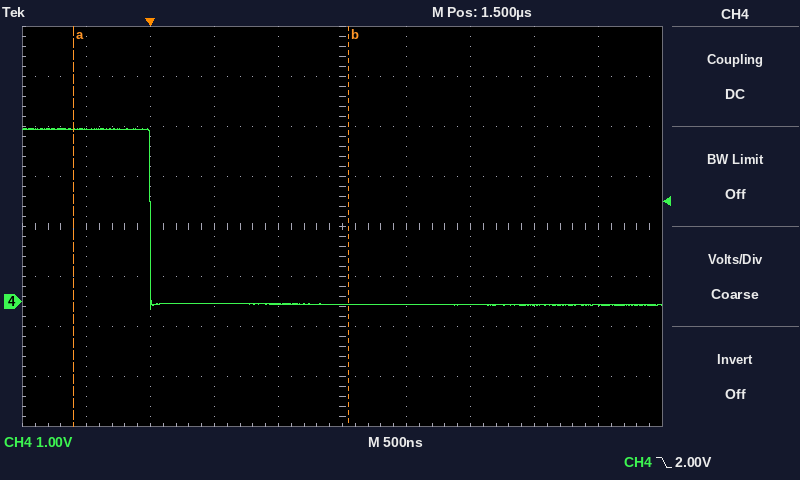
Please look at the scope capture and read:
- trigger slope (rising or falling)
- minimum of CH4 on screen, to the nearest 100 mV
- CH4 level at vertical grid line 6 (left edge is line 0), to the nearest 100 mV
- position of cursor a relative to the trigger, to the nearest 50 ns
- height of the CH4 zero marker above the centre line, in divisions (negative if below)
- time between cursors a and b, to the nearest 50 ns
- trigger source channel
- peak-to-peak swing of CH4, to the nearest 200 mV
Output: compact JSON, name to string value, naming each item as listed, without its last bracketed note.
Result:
{"trigger slope": "falling", "minimum of CH4 on screen, to the nearest 100 mV": "-200 mV", "CH4 level at vertical grid line 6 (left edge is line 0), to the nearest 100 mV": "-100 mV", "position of cursor a relative to the trigger, to the nearest 50 ns": "-600 ns", "height of the CH4 zero marker above the centre line, in divisions": "-1.5 div", "time between cursors a and b, to the nearest 50 ns": "2.15 µs", "trigger source channel": "CH4", "peak-to-peak swing of CH4, to the nearest 200 mV": "3.6 V"}
